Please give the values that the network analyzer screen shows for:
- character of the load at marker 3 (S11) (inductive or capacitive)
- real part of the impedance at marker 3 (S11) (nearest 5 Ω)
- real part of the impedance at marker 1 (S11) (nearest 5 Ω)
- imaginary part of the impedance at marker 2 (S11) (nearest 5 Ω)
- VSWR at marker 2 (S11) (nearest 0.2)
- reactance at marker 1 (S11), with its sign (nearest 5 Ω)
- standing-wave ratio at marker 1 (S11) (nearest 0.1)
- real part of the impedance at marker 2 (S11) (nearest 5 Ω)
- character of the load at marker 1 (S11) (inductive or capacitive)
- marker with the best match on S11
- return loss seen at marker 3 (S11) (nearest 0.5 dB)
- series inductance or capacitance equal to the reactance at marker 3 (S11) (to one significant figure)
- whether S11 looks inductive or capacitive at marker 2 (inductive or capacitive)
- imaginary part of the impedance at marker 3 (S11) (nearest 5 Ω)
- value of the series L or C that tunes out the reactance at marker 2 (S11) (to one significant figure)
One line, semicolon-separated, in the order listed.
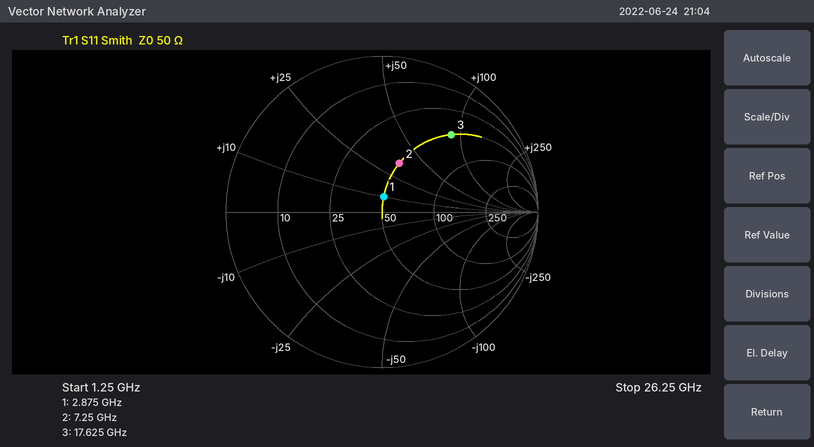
inductive; 50 Ω; 50 Ω; +35 Ω; 2.0; +10 Ω; 1.2; 50 Ω; inductive; marker 1; 3.5 dB; 800 pH; inductive; +90 Ω; 600 fF
